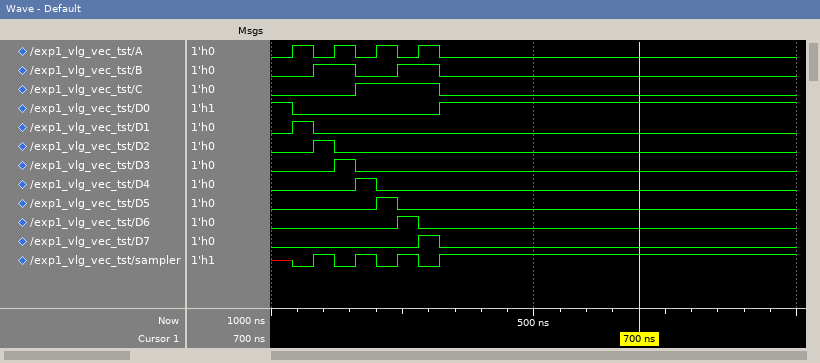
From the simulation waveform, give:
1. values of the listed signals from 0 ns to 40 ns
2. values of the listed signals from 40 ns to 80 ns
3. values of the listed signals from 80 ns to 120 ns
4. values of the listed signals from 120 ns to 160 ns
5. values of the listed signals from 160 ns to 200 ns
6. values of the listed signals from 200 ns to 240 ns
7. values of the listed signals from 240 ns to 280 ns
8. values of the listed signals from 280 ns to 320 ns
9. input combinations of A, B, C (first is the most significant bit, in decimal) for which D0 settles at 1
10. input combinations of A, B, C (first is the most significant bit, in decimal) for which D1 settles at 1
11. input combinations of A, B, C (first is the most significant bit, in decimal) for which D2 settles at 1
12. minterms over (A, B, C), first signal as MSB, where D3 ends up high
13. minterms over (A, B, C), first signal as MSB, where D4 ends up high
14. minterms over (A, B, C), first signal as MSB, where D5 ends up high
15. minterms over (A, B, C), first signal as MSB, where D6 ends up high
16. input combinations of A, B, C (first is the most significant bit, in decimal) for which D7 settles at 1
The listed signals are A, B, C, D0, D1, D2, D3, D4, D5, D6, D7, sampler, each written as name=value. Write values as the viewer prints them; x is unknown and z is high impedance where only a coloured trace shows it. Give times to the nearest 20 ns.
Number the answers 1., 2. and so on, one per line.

1. A=0, B=0, C=0, D0=1, D1=0, D2=0, D3=0, D4=0, D5=0, D6=0, D7=0, sampler=x
2. A=1, B=0, C=0, D0=0, D1=1, D2=0, D3=0, D4=0, D5=0, D6=0, D7=0, sampler=0
3. A=0, B=1, C=0, D0=0, D1=0, D2=1, D3=0, D4=0, D5=0, D6=0, D7=0, sampler=1
4. A=1, B=1, C=0, D0=0, D1=0, D2=0, D3=1, D4=0, D5=0, D6=0, D7=0, sampler=0
5. A=0, B=0, C=1, D0=0, D1=0, D2=0, D3=0, D4=1, D5=0, D6=0, D7=0, sampler=1
6. A=1, B=0, C=1, D0=0, D1=0, D2=0, D3=0, D4=0, D5=1, D6=0, D7=0, sampler=0
7. A=0, B=1, C=1, D0=0, D1=0, D2=0, D3=0, D4=0, D5=0, D6=1, D7=0, sampler=1
8. A=1, B=1, C=1, D0=0, D1=0, D2=0, D3=0, D4=0, D5=0, D6=0, D7=1, sampler=0
9. 0
10. 4
11. 2
12. 6
13. 1
14. 5
15. 3
16. 7
